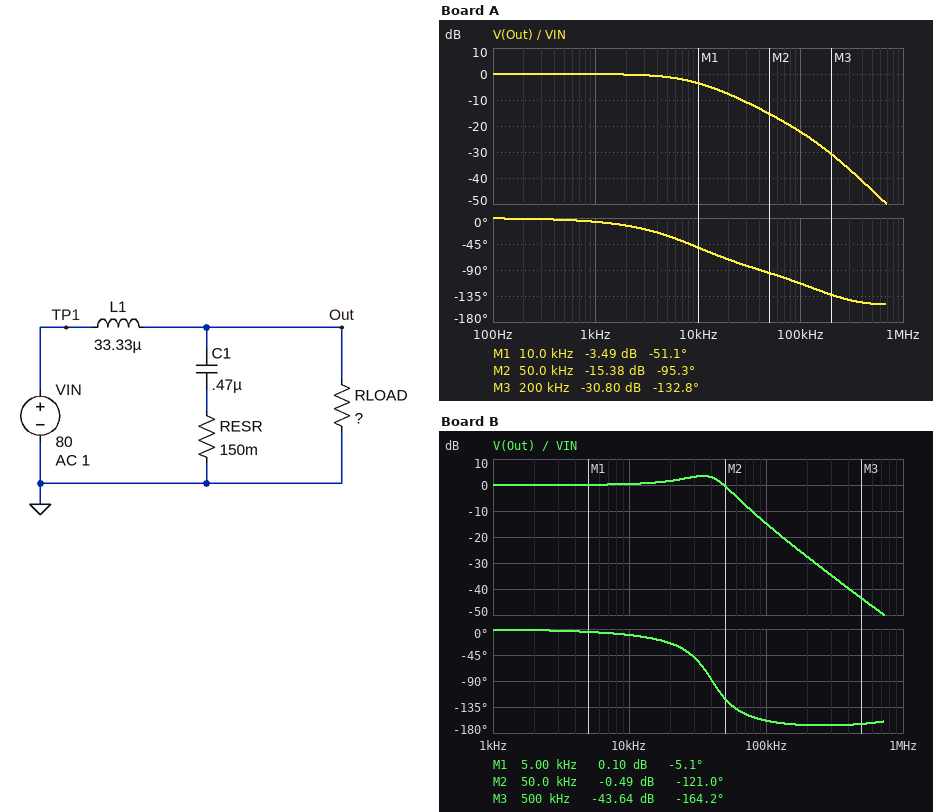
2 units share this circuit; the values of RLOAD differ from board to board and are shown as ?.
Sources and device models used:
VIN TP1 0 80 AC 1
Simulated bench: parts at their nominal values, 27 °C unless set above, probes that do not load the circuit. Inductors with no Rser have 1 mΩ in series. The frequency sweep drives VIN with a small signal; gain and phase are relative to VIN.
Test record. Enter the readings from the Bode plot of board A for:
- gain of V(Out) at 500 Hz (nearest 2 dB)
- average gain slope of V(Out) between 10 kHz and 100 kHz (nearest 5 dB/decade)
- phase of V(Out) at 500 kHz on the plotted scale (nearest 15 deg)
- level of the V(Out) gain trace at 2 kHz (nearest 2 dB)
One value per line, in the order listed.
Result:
0 dB
-20 dB/decade
-150 deg
0 dB
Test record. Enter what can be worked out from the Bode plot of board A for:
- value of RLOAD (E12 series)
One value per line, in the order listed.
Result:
1.8 Ω
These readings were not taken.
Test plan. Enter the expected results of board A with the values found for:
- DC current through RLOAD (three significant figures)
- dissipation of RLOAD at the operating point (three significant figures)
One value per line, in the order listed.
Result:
44.4 A
3.55 kW
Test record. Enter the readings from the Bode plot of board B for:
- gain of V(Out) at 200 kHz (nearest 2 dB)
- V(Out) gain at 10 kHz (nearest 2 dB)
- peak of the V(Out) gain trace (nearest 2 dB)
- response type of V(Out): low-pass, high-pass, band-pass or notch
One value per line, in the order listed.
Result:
-28 dB
0 dB
4 dB
low-pass
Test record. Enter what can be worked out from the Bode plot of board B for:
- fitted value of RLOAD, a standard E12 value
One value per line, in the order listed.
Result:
12 Ω
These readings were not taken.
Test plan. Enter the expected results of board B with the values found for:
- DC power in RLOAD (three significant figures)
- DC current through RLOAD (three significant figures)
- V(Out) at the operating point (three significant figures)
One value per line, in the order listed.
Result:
533 W
6.67 A
80.0 V
